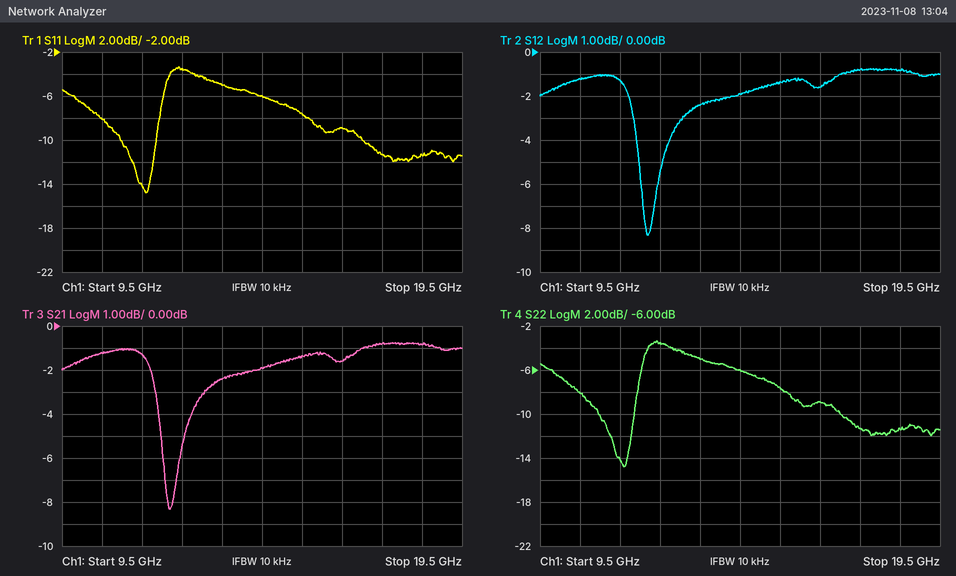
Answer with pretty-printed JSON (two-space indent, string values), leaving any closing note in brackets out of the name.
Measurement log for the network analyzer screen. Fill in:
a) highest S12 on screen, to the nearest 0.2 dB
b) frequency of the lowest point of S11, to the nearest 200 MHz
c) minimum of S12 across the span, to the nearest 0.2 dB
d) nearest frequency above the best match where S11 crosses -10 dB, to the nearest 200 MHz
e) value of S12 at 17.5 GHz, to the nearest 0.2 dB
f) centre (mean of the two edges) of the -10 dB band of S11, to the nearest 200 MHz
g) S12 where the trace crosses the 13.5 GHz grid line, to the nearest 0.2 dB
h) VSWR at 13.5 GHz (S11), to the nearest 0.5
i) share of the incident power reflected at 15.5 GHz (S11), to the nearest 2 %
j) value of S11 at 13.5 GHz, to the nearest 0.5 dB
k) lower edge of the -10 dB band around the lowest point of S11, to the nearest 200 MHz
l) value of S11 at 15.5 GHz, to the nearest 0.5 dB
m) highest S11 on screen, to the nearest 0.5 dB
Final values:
{
  "highest S12 on screen, to the nearest 0.2 dB": "-0.8 dB",
  "frequency of the lowest point of S11, to the nearest 200 MHz": "11.6 GHz",
  "minimum of S12 across the span, to the nearest 0.2 dB": "-8.4 dB",
  "nearest frequency above the best match where S11 crosses -10 dB, to the nearest 200 MHz": "11.8 GHz",
  "value of S12 at 17.5 GHz, to the nearest 0.2 dB": "-0.8 dB",
  "centre (mean of the two edges) of the -10 dB band of S11, to the nearest 200 MHz": "11.4 GHz",
  "S12 where the trace crosses the 13.5 GHz grid line, to the nearest 0.2 dB": "-2.4 dB",
  "VSWR at 13.5 GHz (S11), to the nearest 0.5": "3.5",
  "share of the incident power reflected at 15.5 GHz (S11), to the nearest 2 %": "18 %",
  "value of S11 at 13.5 GHz, to the nearest 0.5 dB": "-5.0 dB",
  "lower edge of the -10 dB band around the lowest point of S11, to the nearest 200 MHz": "11.0 GHz",
  "value of S11 at 15.5 GHz, to the nearest 0.5 dB": "-7.5 dB",
  "highest S11 on screen, to the nearest 0.5 dB": "-3.5 dB"
}
